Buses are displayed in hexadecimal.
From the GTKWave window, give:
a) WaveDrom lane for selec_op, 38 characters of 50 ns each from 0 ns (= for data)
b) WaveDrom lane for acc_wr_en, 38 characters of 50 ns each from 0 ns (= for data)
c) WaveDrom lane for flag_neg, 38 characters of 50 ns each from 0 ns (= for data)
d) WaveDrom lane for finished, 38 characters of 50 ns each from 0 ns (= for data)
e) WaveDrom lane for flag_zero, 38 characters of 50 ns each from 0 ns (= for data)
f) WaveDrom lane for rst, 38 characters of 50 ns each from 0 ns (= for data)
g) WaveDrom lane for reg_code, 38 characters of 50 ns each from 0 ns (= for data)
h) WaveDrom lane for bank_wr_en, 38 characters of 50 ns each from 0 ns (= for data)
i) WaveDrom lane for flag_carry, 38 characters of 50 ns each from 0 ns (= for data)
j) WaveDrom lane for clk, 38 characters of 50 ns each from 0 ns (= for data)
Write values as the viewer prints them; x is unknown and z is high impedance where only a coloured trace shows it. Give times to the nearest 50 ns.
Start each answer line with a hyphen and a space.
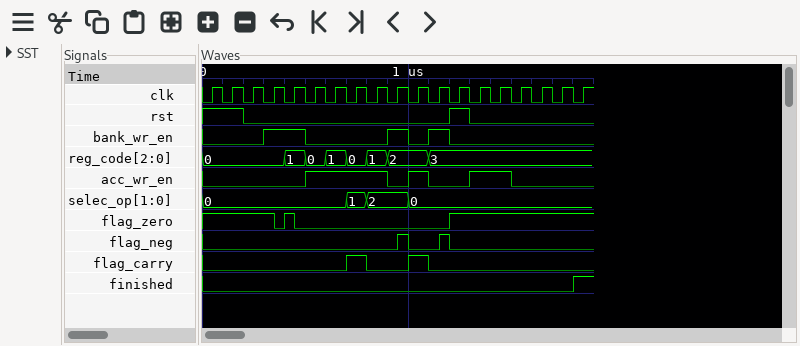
- {name: 'selec_op', wave: '=.............=.=...=.................', data: '0 1 2 0'}
- {name: 'acc_wr_en', wave: '0.........1.......0.1.0...1...0.......'}
- {name: 'flag_neg', wave: '0..................10..10.............'}
- {name: 'finished', wave: '0...................................1.'}
- {name: 'flag_zero', wave: '1......010..............1.............'}
- {name: 'rst', wave: '1...0...................1.0...........'}
- {name: 'reg_code', wave: '=.......=.=.=.=.=.=...=...............', data: '0 1 0 1 0 1 2 3'}
- {name: 'bank_wr_en', wave: '0.....1...0.......1.0.1.0.............'}
- {name: 'flag_carry', wave: '0.............1.0...1.0...............'}
- {name: 'clk', wave: '01010101010101010101010101010101010101'}
